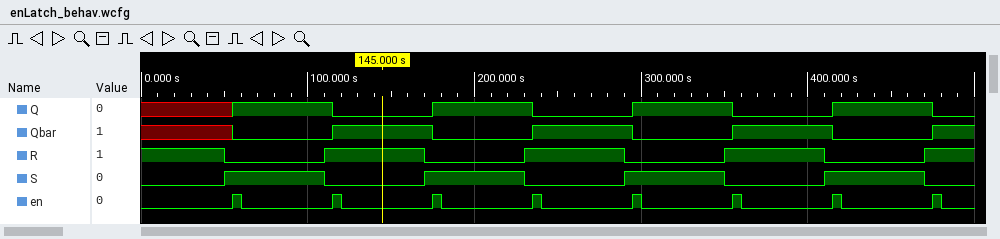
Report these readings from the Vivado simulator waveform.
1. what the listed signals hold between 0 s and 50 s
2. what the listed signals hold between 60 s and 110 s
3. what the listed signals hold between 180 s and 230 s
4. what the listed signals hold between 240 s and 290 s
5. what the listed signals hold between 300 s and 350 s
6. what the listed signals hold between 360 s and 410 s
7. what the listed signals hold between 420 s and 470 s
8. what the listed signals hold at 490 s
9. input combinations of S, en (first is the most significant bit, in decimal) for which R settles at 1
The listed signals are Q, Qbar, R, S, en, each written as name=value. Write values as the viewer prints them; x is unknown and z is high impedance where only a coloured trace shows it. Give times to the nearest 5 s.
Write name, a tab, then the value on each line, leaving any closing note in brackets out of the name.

what the listed signals hold between 0 s and 50 s	Q=x, Qbar=x, R=1, S=0, en=0
what the listed signals hold between 60 s and 110 s	Q=1, Qbar=0, R=0, S=1, en=0
what the listed signals hold between 180 s and 230 s	Q=1, Qbar=0, R=0, S=1, en=0
what the listed signals hold between 240 s and 290 s	Q=0, Qbar=1, R=1, S=0, en=0
what the listed signals hold between 300 s and 350 s	Q=1, Qbar=0, R=0, S=1, en=0
what the listed signals hold between 360 s and 410 s	Q=0, Qbar=1, R=1, S=0, en=0
what the listed signals hold between 420 s and 470 s	Q=1, Qbar=0, R=0, S=1, en=0
what the listed signals hold at 490 s	Q=0, Qbar=1, R=1, S=0, en=0
input combinations of S, en (first is the most significant bit, in decimal) for which R settles at 1	0, 1
